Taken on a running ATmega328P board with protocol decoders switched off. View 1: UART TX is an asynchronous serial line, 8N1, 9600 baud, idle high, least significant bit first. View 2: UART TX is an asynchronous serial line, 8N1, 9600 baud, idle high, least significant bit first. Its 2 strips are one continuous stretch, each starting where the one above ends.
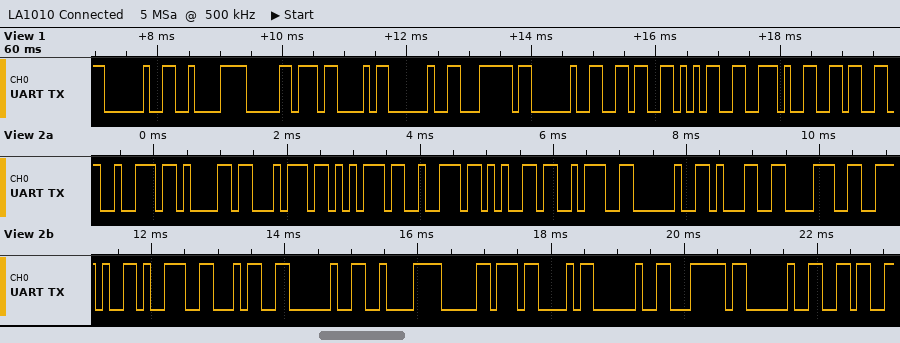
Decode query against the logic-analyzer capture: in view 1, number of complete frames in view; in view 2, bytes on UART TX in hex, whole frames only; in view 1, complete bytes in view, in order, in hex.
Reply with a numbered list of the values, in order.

1. 11
2. 0x72 0x61 0x74 0x75 0x72 0x65 0x3A 0x20 0x31 0x38 0x2E 0x39 0x34 0x20 0xC2 0xB0 0x43 0x20 0x7C 0x20 0x36
3. 20 C2 B0 43 20 7C 20 36 35 2E 36
